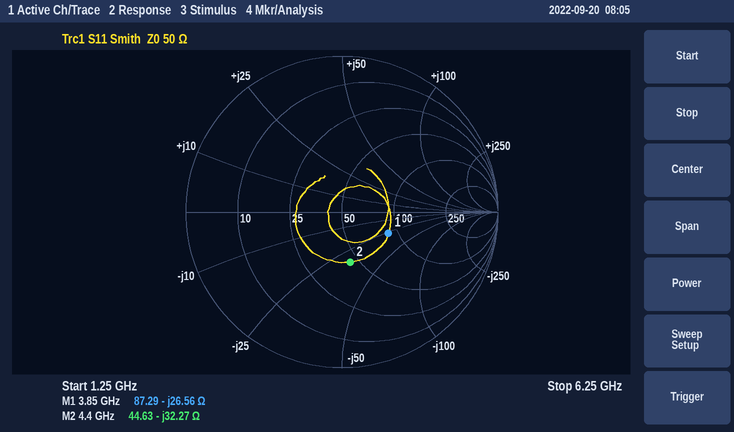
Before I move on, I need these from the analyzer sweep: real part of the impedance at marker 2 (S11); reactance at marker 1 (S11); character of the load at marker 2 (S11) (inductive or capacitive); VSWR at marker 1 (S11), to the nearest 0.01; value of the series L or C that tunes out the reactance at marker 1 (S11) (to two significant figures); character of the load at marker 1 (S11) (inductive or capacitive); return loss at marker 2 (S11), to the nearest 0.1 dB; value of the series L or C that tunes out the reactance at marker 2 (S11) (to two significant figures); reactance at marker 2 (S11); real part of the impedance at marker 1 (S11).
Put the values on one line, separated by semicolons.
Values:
44.63 Ω; -26.56 Ω; capacitive; 1.97; 1.1 nH; capacitive; 9.7 dB; 1.2 nH; -32.27 Ω; 87.29 Ω
